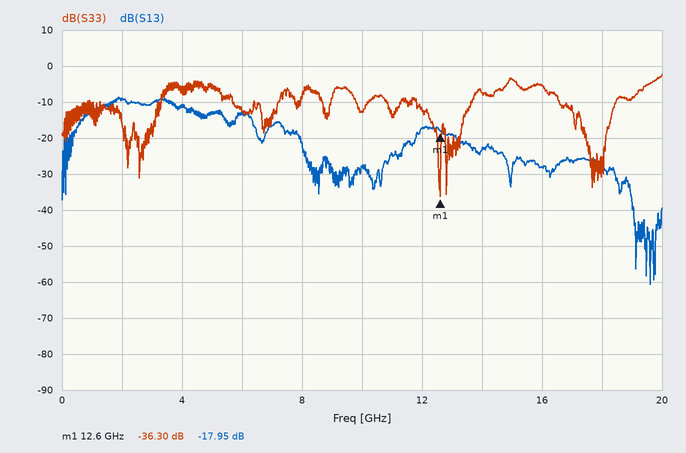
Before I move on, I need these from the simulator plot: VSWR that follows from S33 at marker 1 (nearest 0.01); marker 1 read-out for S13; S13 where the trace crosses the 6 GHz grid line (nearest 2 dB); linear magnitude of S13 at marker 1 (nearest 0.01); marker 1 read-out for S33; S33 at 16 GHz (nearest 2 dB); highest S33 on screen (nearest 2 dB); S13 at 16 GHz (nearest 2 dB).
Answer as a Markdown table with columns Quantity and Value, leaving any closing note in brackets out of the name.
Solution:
| Quantity | Value |
|---|---|
| VSWR that follows from S33 at marker 1 | 1.03 |
| marker 1 read-out for S13 | -17.95 dB |
| S13 where the trace crosses the 6 GHz grid line | -14 dB |
| linear magnitude of S13 at marker 1 | 0.13 |
| marker 1 read-out for S33 | -36.30 dB |
| S33 at 16 GHz | -6 dB |
| highest S33 on screen | -2 dB |
| S13 at 16 GHz | -28 dB |
